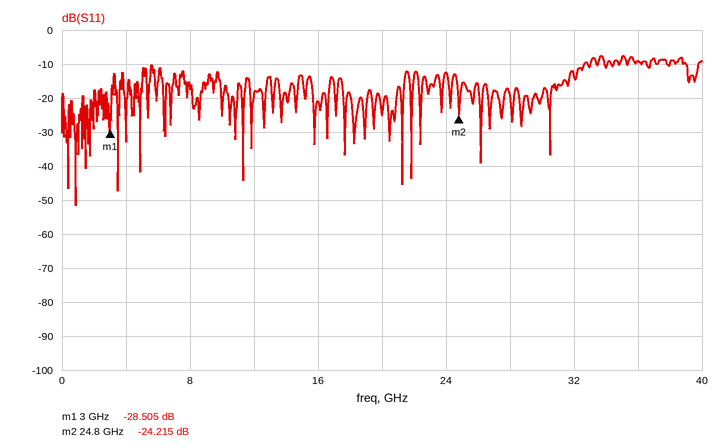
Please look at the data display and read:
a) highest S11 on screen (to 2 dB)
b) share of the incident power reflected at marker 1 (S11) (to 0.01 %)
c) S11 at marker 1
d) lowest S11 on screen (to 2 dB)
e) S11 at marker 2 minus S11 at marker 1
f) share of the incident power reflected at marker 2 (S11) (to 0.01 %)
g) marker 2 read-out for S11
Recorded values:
-8 dB
0.14 %
-28.505 dB
-52 dB
4.290 dB
0.38 %
-24.215 dB
